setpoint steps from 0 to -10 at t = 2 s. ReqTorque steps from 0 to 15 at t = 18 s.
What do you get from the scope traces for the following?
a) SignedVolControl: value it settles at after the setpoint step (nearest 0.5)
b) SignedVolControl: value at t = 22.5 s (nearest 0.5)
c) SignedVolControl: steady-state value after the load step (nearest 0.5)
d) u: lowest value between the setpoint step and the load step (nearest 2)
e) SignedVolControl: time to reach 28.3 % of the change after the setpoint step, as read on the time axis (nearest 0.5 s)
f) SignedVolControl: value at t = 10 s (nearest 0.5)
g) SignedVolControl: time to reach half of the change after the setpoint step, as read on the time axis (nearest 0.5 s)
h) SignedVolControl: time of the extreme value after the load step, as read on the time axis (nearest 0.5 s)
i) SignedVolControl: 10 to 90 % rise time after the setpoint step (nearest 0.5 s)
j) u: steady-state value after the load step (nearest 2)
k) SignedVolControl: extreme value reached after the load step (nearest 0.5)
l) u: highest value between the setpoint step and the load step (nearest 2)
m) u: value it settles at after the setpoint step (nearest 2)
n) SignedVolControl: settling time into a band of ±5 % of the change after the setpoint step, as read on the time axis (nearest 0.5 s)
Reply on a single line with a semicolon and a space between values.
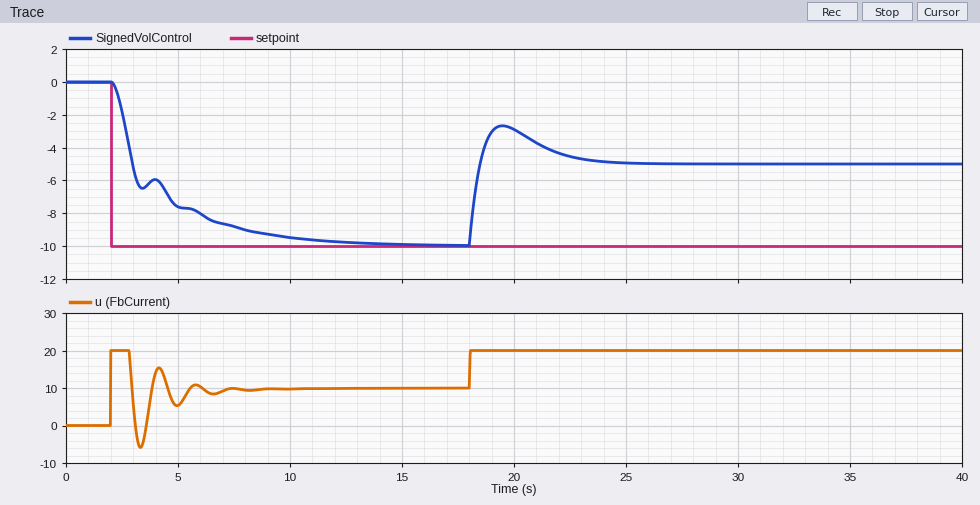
-10.0; -4.5; -5.0; -6; 2.5 s; -9.5; 3.0 s; 19.5 s; 5.5 s; 20; -2.5; 20; 10; 10.0 s
